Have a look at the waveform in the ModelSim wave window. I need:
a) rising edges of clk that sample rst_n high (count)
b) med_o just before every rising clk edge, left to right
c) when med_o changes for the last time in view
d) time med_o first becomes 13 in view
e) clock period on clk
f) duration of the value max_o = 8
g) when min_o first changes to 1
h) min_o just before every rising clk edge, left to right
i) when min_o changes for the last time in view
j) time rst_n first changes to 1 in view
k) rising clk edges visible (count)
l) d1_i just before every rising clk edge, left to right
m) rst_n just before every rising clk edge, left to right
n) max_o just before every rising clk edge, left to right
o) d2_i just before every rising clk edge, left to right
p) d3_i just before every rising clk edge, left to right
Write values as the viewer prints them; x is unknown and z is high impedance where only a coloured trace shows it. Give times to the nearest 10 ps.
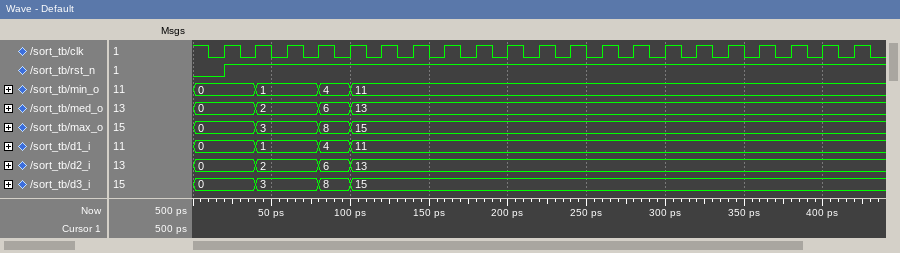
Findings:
20
0, 0, 2, 2, 6, 13, 13, 13, 13, 13, 13, 13, 13, 13, 13, 13, 13, 13, 13, 13, 13
100 ps
100 ps
20 ps
20 ps
40 ps
0, 0, 1, 1, 4, 11, 11, 11, 11, 11, 11, 11, 11, 11, 11, 11, 11, 11, 11, 11, 11
100 ps
20 ps
21
0, 0, 1, 1, 4, 11, 11, 11, 11, 11, 11, 11, 11, 11, 11, 11, 11, 11, 11, 11, 11
0 1 1 1 1 1 1 1 1 1 1 1 1 1 1 1 1 1 1 1 1
0, 0, 3, 3, 8, 15, 15, 15, 15, 15, 15, 15, 15, 15, 15, 15, 15, 15, 15, 15, 15
0, 0, 2, 2, 6, 13, 13, 13, 13, 13, 13, 13, 13, 13, 13, 13, 13, 13, 13, 13, 13
0, 0, 3, 3, 8, 15, 15, 15, 15, 15, 15, 15, 15, 15, 15, 15, 15, 15, 15, 15, 15
